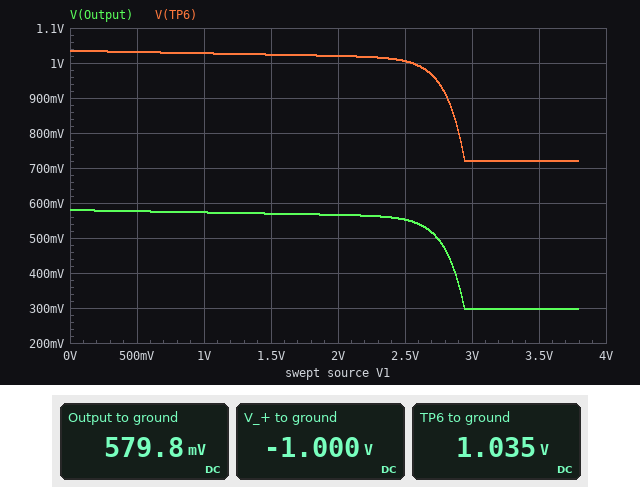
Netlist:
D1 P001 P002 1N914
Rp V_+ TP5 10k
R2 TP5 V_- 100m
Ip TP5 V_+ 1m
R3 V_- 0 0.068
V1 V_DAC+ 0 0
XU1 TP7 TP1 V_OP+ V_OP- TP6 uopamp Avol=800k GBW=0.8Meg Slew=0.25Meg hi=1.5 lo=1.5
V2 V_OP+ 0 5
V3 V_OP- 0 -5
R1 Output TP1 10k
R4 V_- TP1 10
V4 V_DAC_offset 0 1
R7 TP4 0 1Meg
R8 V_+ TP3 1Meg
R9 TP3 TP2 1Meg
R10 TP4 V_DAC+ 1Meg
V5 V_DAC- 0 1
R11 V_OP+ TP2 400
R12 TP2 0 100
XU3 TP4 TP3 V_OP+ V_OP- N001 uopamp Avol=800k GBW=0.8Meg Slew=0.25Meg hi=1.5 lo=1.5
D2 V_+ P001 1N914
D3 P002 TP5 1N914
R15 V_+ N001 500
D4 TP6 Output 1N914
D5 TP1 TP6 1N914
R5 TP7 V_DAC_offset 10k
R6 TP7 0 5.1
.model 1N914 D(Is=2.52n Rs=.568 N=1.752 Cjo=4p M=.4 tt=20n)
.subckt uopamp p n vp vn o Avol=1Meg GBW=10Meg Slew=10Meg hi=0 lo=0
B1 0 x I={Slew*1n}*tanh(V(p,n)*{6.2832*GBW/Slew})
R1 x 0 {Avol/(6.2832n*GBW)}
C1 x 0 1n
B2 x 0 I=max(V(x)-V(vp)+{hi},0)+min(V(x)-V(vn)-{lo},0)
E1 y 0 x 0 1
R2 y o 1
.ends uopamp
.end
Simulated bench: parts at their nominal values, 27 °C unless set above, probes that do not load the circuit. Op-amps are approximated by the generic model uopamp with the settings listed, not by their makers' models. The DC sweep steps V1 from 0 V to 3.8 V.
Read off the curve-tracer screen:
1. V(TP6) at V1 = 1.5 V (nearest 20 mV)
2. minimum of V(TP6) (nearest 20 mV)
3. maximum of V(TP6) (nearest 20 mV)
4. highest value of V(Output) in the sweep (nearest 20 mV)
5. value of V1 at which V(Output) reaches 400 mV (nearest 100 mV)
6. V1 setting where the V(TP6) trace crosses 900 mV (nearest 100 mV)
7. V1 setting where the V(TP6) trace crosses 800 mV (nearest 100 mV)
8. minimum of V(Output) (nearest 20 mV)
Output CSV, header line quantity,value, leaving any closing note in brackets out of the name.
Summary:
quantity,value
V(TP6) at V1 = 1.5 V,1.02 V
minimum of V(TP6),720 mV
maximum of V(TP6),1.04 V
highest value of V(Output) in the sweep,580 mV
value of V1 at which V(Output) reaches 400 mV,2.9 V
V1 setting where the V(TP6) trace crosses 900 mV,2.8 V
V1 setting where the V(TP6) trace crosses 800 mV,2.9 V
minimum of V(Output),300 mV
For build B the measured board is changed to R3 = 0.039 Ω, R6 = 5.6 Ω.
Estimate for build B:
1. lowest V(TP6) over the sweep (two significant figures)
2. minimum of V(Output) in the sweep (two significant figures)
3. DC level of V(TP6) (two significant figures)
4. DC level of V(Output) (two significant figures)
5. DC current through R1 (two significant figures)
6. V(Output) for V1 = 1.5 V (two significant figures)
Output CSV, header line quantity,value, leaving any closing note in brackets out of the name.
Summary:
quantity,value
lowest V(TP6) over the sweep,880 mV
minimum of V(Output) in the sweep,440 mV
DC level of V(TP6),1.1 V
DC level of V(Output),600 mV
DC current through R1,60 µA
V(Output) for V1 = 1.5 V,590 mV
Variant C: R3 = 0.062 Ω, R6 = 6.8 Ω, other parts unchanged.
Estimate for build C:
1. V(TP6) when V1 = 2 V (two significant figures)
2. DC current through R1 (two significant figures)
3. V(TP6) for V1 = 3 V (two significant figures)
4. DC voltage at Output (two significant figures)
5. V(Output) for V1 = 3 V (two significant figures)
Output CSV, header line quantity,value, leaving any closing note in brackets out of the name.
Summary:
quantity,value
V(TP6) when V1 = 2 V,1.2 V
DC current through R1,74 µA
V(TP6) for V1 = 3 V,930 mV
DC voltage at Output,740 mV
V(Output) for V1 = 3 V,480 mV
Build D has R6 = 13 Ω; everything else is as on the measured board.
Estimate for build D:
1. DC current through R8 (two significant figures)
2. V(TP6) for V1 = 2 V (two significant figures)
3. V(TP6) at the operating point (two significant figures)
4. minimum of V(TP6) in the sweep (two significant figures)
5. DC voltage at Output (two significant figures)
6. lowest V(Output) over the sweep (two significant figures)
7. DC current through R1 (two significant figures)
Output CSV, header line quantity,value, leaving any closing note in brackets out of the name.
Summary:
quantity,value
DC current through R8,1.0 µA
V(TP6) for V1 = 2 V,1.8 V
V(TP6) at the operating point,1.9 V
minimum of V(TP6) in the sweep,1.6 V
DC voltage at Output,1.4 V
lowest V(Output) over the sweep,1.1 V
DC current through R1,140 µA
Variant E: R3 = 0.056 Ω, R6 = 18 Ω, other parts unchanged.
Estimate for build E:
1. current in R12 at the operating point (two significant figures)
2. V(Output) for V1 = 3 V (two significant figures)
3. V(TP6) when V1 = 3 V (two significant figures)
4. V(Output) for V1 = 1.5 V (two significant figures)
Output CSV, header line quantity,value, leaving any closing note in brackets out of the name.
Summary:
quantity,value
current in R12 at the operating point,10 mA
V(Output) for V1 = 3 V,1.6 V
V(TP6) when V1 = 3 V,2.1 V
V(Output) for V1 = 1.5 V,1.8 V
